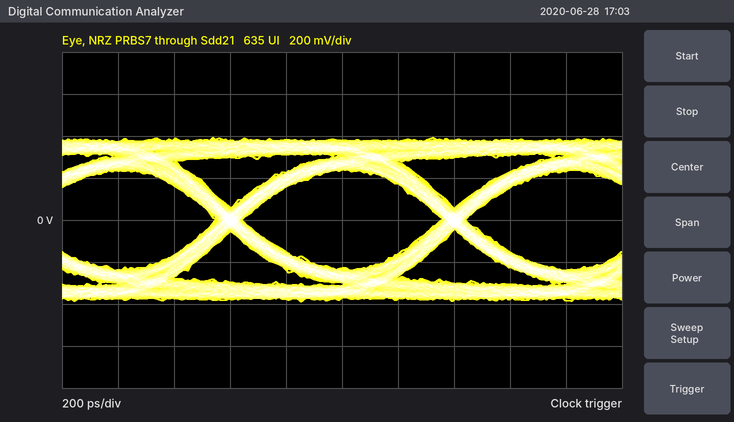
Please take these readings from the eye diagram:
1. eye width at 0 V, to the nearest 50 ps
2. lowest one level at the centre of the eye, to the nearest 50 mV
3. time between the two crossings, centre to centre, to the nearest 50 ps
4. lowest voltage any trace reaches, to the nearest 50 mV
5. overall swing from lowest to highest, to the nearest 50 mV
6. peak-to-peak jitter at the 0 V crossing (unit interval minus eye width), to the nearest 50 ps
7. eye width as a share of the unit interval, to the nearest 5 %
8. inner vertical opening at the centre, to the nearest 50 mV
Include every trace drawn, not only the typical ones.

700 ps
250 mV
800 ps
-400 mV
800 mV
100 ps
90 %
450 mV
